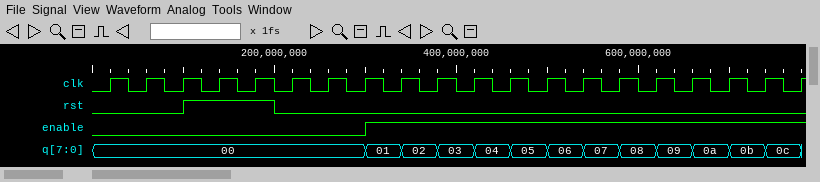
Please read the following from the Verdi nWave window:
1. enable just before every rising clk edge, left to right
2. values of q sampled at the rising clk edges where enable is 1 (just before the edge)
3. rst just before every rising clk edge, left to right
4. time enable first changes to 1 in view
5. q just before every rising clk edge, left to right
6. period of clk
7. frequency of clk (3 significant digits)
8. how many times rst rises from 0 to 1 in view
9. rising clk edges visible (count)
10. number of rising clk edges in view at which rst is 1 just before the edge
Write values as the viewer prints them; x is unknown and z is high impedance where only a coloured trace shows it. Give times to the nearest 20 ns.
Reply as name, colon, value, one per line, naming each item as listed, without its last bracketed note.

enable just before every rising clk edge, left to right: 0 0 0 0 0 0 0 0 1 1 1 1 1 1 1 1 1 1 1 1
values of q sampled at the rising clk edges where enable is 1: 01, 02, 03, 04, 05, 06, 07, 08, 09, 0a, 0b, 0c
rst just before every rising clk edge, left to right: 0 0 0 1 1 0 0 0 0 0 0 0 0 0 0 0 0 0 0 0
time enable first changes to 1 in view: 300 ns
q just before every rising clk edge, left to right: 00, 00, 00, 00, 00, 00, 00, 00, 01, 02, 03, 04, 05, 06, 07, 08, 09, 0a, 0b, 0c
period of clk: 40 ns
frequency of clk: 25.0 MHz
how many times rst rises from 0 to 1 in view: 1
rising clk edges visible: 20
number of rising clk edges in view at which rst is 1 just before the edge: 2
